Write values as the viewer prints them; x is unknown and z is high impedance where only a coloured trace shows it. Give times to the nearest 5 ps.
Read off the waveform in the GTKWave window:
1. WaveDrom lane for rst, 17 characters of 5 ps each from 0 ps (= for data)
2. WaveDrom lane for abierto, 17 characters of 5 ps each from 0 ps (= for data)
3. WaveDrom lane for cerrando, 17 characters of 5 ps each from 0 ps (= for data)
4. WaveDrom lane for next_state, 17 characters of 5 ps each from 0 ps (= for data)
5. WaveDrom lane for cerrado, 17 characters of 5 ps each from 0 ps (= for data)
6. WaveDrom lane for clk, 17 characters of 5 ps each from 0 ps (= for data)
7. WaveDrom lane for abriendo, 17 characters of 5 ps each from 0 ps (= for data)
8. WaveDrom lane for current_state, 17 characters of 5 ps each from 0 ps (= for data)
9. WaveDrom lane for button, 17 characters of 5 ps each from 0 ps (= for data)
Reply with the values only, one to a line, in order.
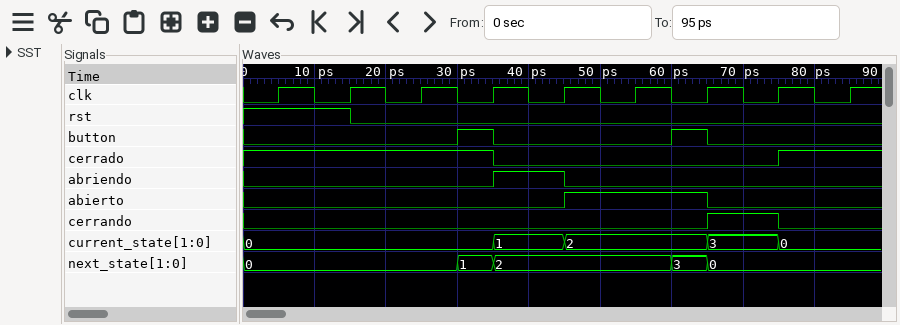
{name: 'rst', wave: '1..0.............'}
{name: 'abierto', wave: '0........1...0...'}
{name: 'cerrando', wave: '0............1.0.'}
{name: 'next_state', wave: '=.....==....==...', data: '0 1 2 3 0'}
{name: 'cerrado', wave: '1......0.......1.'}
{name: 'clk', wave: '01010101010101010'}
{name: 'abriendo', wave: '0......1.0.......'}
{name: 'current_state', wave: '=......=.=...=.=.', data: '0 1 2 3 0'}
{name: 'button', wave: '0.....10....10...'}
